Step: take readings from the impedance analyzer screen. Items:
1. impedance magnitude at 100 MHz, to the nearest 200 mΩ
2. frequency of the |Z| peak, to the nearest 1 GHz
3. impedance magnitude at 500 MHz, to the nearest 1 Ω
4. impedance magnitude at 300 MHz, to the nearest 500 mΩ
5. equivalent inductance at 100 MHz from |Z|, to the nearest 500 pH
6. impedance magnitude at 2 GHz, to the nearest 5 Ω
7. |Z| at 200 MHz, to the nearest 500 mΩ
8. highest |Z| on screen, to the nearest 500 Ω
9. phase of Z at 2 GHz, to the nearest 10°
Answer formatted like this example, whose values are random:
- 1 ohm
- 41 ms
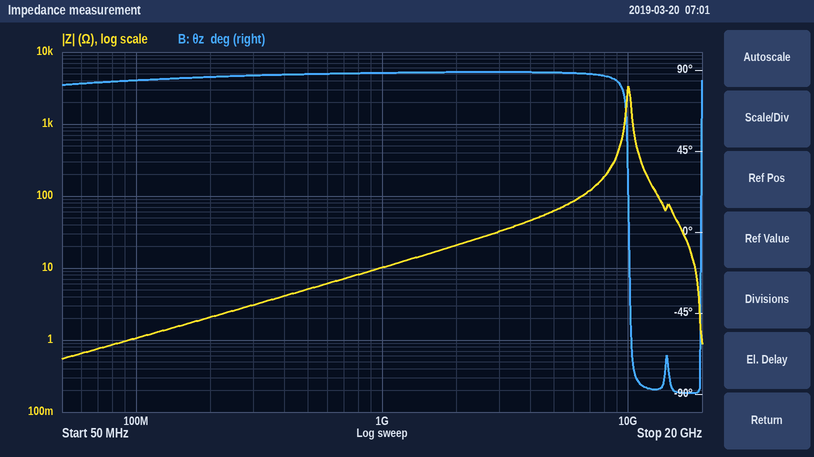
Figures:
- 1.0 Ω
- 10 GHz
- 5 Ω
- 3.0 Ω
- 1.5 nH
- 20 Ω
- 2.0 Ω
- 3.5 kΩ
- 90°
